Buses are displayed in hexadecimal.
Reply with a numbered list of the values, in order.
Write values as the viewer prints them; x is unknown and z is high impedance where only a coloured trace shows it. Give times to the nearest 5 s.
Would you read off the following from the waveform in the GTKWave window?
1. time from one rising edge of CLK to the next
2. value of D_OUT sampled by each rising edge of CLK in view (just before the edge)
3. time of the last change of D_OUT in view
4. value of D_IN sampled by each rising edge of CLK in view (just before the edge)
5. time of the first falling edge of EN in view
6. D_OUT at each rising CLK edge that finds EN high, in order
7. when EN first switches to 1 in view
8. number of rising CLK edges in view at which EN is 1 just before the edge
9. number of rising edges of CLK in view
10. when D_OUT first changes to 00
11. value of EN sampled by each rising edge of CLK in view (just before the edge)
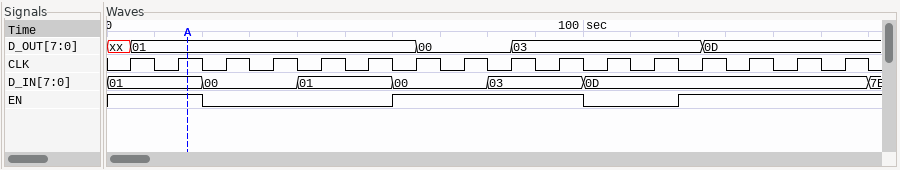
1. 10 s
2. xx, 01, 01, 01, 01, 01, 01, 00, 00, 03, 03, 03, 03, 0D, 0D, 0D
3. 125 s
4. 01, 01, 00, 00, 01, 01, 00, 00, 03, 03, 0D, 0D, 0D, 0D, 0D, 0D
5. 20 s
6. xx, 01, 01, 00, 00, 03, 03, 0D, 0D, 0D
7. 60 s
8. 10
9. 16
10. 65 s
11. 1 1 0 0 0 0 1 1 1 1 0 0 1 1 1 1
